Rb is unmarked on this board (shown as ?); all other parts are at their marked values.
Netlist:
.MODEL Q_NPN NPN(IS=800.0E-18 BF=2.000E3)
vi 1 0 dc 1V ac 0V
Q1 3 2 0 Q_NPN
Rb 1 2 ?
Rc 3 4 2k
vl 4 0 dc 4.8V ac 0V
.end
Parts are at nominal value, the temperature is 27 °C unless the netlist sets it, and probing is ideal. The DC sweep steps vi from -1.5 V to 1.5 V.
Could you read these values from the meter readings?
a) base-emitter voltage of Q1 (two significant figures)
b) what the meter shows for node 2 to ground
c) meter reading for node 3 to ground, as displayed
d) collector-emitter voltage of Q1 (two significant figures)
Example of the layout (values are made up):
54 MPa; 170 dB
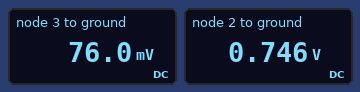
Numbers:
750 mV; 0.746 V; 76.0 mV; 76 mV
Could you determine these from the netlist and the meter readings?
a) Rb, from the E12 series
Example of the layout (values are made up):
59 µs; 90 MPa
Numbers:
1.8 kΩ
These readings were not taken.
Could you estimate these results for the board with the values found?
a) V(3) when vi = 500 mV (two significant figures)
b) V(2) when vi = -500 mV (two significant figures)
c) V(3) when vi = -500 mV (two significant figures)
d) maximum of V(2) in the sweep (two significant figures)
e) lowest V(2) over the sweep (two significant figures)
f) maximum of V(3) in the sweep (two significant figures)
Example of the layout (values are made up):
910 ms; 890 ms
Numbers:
4.8 V; -500 mV; 4.8 V; 750 mV; -1.5 V; 4.8 V
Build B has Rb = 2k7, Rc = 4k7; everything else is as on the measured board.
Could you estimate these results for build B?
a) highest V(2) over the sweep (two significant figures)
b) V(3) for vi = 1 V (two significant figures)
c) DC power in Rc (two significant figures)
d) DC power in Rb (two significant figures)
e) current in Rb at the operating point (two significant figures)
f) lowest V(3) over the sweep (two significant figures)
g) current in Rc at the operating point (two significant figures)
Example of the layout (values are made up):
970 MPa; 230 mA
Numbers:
730 mV; 64 mV; 4.8 mW; 28 µW; 100 µA; 44 mV; 1.0 mA
